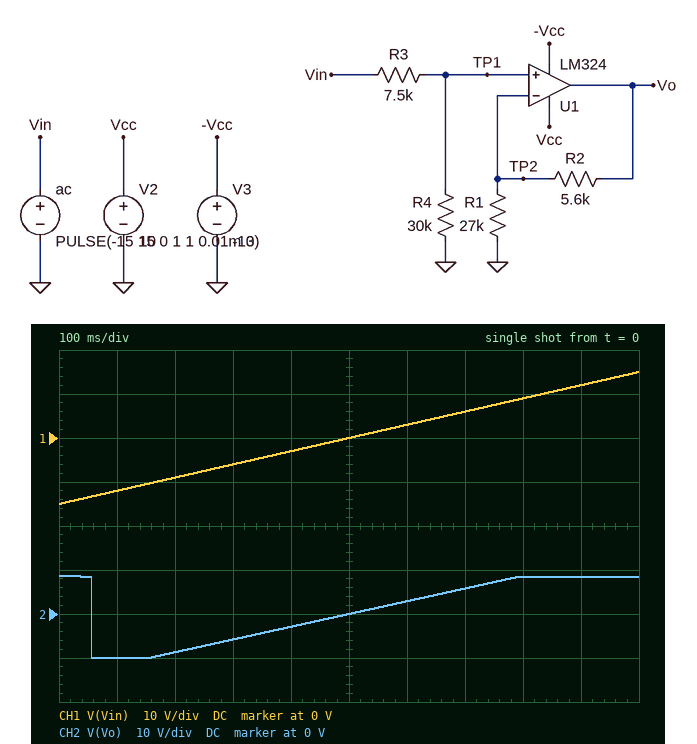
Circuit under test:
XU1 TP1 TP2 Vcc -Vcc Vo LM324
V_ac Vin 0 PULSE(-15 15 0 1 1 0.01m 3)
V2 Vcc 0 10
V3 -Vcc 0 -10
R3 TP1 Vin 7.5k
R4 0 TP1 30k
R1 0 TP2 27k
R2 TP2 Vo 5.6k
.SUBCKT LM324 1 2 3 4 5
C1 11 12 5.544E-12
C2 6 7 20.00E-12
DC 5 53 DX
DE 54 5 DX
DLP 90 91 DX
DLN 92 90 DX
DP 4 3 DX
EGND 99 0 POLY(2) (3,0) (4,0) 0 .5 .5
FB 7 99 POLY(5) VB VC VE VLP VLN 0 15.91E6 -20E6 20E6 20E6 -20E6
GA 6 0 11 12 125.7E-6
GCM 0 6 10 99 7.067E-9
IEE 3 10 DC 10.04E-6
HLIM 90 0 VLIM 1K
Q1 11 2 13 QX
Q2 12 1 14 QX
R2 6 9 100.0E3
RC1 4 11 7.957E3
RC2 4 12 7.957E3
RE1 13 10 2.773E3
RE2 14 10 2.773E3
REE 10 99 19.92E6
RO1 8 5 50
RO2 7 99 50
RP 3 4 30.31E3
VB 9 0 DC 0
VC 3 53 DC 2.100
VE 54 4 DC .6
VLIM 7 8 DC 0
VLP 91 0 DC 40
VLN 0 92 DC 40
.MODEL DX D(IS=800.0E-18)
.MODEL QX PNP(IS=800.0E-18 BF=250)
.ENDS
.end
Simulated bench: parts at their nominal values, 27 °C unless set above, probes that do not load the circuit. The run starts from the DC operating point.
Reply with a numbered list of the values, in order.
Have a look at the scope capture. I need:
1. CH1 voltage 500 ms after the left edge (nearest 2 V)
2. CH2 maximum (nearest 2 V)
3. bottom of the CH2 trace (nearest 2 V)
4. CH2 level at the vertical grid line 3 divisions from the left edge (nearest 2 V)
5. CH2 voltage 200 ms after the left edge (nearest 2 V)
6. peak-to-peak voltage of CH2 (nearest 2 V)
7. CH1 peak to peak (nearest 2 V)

1. 0 V
2. 8 V
3. -10 V
4. -6 V
5. -8 V
6. 18 V
7. 30 V
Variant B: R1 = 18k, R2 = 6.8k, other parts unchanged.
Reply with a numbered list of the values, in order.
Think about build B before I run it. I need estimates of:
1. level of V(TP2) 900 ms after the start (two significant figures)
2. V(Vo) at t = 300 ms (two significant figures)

1. 6.2 V
2. -6.6 V
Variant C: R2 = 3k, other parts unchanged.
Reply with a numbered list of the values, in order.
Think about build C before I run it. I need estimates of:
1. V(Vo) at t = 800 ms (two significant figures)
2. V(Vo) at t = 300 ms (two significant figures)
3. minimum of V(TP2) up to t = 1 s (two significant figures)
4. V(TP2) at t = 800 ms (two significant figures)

1. 8.0 V
2. -5.3 V
3. -9.0 V
4. 7.2 V
